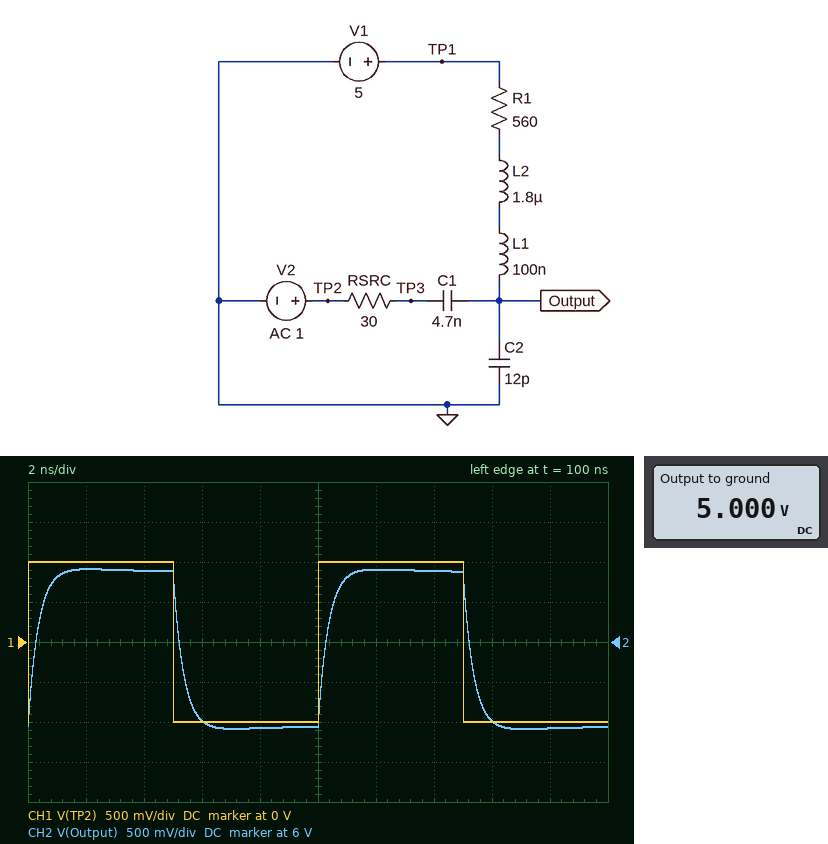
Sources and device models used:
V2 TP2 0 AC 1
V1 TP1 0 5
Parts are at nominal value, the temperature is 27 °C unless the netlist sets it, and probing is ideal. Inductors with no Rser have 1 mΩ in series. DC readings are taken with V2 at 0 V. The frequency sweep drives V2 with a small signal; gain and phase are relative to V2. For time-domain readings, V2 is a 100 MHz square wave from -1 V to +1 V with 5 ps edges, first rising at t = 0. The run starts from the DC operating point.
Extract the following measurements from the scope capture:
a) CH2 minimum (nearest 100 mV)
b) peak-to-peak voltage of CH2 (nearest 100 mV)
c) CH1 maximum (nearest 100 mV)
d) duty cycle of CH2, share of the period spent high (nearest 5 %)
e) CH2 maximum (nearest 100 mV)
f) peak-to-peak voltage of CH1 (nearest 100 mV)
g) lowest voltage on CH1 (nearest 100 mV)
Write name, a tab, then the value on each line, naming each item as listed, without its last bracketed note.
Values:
CH2 minimum	4.9 V
peak-to-peak voltage of CH2	2.0 V
CH1 maximum	1.0 V
duty cycle of CH2, share of the period spent high	50 %
CH2 maximum	6.9 V
peak-to-peak voltage of CH1	2.0 V
lowest voltage on CH1	-1.0 V
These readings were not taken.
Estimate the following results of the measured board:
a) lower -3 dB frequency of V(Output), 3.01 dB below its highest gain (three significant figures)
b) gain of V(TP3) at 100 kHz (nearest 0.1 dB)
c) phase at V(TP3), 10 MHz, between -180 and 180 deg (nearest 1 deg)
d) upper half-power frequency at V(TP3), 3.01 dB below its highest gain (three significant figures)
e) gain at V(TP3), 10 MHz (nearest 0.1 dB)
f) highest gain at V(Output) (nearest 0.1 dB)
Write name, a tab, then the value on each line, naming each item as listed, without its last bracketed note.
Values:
lower -3 dB frequency of V(Output), 3.01 dB below its highest gain	60.5 kHz
gain of V(TP3) at 100 kHz	-0.3 dB
phase at V(TP3), 10 MHz, between -180 and 180 deg	-1 deg
upper half-power frequency at V(TP3), 3.01 dB below its highest gain	445 MHz
gain at V(TP3), 10 MHz	-0.4 dB
highest gain at V(Output)	-0.2 dB
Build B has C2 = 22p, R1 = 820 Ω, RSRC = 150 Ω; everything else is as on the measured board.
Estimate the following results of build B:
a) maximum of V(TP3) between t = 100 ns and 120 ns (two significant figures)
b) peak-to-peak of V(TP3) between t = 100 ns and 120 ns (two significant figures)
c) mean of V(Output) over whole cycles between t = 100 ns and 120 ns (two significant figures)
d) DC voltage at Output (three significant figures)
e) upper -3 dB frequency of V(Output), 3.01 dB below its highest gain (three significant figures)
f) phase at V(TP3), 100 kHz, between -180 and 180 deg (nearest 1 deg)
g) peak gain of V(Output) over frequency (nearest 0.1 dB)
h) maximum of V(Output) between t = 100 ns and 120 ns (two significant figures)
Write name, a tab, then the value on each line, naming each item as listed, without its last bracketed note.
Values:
maximum of V(TP3) between t = 100 ns and 120 ns	490 mV
peak-to-peak of V(TP3) between t = 100 ns and 120 ns	1.3 V
mean of V(Output) over whole cycles between t = 100 ns and 120 ns	5.8 V
DC voltage at Output	5.00 V
upper -3 dB frequency of V(Output), 3.01 dB below its highest gain	65.6 MHz
phase at V(TP3), 100 kHz, between -180 and 180 deg	-3 deg
peak gain of V(Output) over frequency	-1.5 dB
maximum of V(Output) between t = 100 ns and 120 ns	6.5 V
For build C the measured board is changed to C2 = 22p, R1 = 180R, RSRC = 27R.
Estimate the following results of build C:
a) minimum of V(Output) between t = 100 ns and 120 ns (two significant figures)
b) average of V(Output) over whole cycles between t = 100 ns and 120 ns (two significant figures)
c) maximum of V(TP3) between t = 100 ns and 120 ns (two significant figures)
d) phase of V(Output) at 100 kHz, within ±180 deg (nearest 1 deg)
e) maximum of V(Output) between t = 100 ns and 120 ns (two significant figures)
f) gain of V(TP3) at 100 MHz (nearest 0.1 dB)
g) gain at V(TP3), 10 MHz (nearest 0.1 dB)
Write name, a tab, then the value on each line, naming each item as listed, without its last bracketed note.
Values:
minimum of V(Output) between t = 100 ns and 120 ns	4.8 V
average of V(Output) over whole cycles between t = 100 ns and 120 ns	5.8 V
maximum of V(TP3) between t = 100 ns and 120 ns	880 mV
phase of V(Output) at 100 kHz, within ±180 deg	59 deg
maximum of V(Output) between t = 100 ns and 120 ns	6.8 V
gain of V(TP3) at 100 MHz	-0.5 dB
gain at V(TP3), 10 MHz	-0.9 dB
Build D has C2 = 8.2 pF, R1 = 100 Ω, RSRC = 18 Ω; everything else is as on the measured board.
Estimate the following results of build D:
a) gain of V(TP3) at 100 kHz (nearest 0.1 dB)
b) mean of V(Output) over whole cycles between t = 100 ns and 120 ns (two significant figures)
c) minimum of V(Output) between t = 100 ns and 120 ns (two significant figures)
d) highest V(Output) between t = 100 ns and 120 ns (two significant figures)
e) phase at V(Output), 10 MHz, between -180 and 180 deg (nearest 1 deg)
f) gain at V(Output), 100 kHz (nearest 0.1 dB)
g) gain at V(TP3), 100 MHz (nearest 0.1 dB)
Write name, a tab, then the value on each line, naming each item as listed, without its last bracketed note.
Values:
gain of V(TP3) at 100 kHz	-0.1 dB
mean of V(Output) over whole cycles between t = 100 ns and 120 ns	5.7 V
minimum of V(Output) between t = 100 ns and 120 ns	4.7 V
highest V(Output) between t = 100 ns and 120 ns	6.7 V
phase at V(Output), 10 MHz, between -180 and 180 deg	5 deg
gain at V(Output), 100 kHz	-11.1 dB
gain at V(TP3), 100 MHz	0 dB
